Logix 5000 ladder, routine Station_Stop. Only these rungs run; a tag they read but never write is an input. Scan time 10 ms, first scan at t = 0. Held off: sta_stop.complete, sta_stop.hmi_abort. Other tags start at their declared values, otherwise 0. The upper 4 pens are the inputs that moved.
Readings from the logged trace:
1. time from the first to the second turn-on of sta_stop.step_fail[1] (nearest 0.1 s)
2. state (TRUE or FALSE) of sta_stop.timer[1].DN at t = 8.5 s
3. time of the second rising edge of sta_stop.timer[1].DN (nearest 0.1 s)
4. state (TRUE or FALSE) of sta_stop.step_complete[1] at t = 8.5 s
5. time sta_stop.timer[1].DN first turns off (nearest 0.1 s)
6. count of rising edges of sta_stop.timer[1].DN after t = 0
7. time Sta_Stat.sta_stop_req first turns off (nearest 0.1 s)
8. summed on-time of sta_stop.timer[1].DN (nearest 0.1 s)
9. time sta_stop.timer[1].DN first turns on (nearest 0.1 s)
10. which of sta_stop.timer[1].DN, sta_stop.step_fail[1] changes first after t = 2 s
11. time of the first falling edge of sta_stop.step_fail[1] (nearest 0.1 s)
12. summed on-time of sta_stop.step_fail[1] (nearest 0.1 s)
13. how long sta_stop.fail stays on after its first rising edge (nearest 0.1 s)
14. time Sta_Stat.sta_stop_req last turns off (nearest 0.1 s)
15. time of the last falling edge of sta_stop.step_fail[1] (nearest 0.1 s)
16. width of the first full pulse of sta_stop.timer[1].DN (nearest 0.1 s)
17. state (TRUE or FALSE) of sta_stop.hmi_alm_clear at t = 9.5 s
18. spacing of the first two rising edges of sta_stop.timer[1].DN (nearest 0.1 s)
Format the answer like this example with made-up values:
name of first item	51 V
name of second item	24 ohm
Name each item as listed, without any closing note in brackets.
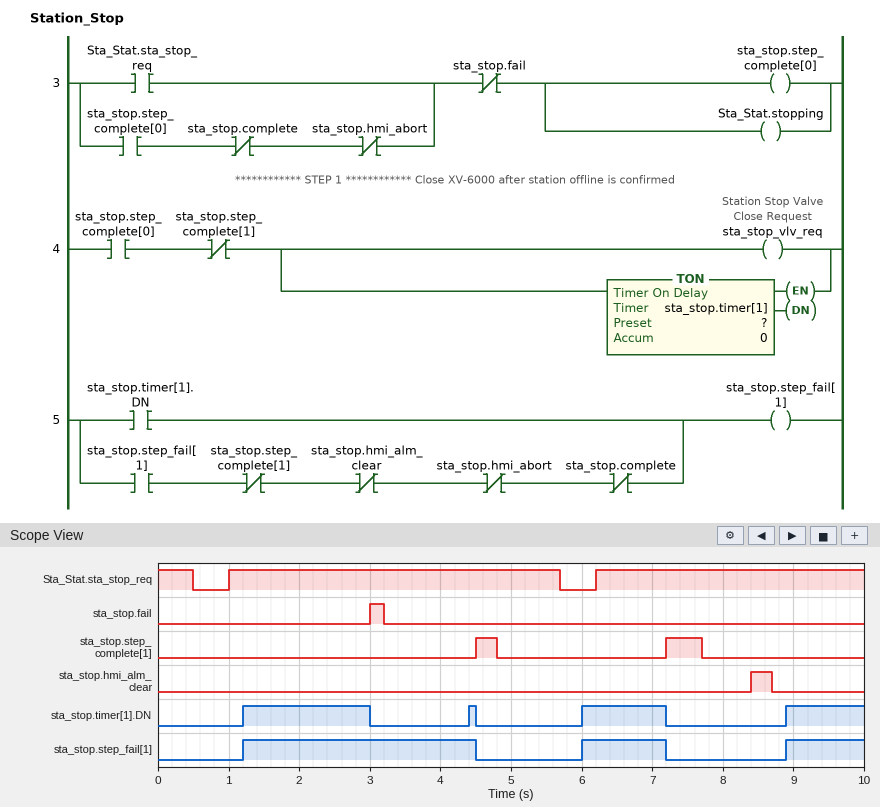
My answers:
time from the first to the second turn-on of sta_stop.step_fail[1]	4.8 s
state (TRUE or FALSE) of sta_stop.timer[1].DN at t = 8.5 s	FALSE
time of the second rising edge of sta_stop.timer[1].DN	4.4 s
state (TRUE or FALSE) of sta_stop.step_complete[1] at t = 8.5 s	FALSE
time sta_stop.timer[1].DN first turns off	3.0 s
count of rising edges of sta_stop.timer[1].DN after t = 0	4
time Sta_Stat.sta_stop_req first turns off	0.5 s
summed on-time of sta_stop.timer[1].DN	4.2 s
time sta_stop.timer[1].DN first turns on	1.2 s
which of sta_stop.timer[1].DN, sta_stop.step_fail[1] changes first after t = 2 s	sta_stop.timer[1].DN
time of the first falling edge of sta_stop.step_fail[1]	4.5 s
summed on-time of sta_stop.step_fail[1]	5.6 s
how long sta_stop.fail stays on after its first rising edge	0.2 s
time Sta_Stat.sta_stop_req last turns off	5.7 s
time of the last falling edge of sta_stop.step_fail[1]	7.2 s
width of the first full pulse of sta_stop.timer[1].DN	1.8 s
state (TRUE or FALSE) of sta_stop.hmi_alm_clear at t = 9.5 s	FALSE
spacing of the first two rising edges of sta_stop.timer[1].DN	3.2 s
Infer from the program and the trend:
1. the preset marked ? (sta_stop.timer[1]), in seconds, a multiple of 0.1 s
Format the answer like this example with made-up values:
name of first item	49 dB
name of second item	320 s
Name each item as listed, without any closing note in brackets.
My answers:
the preset marked ? (sta_stop.timer[1]), in seconds, a multiple of 0.1 s	1.2 s
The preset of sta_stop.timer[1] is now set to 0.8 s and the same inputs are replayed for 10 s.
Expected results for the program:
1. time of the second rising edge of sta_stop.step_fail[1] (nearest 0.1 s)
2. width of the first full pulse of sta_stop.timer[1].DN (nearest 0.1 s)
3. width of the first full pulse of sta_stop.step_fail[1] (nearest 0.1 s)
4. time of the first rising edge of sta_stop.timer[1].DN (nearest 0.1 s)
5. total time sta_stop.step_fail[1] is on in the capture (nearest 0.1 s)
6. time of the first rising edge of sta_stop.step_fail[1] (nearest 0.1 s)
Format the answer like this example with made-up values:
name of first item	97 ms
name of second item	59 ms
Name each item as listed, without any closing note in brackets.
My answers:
time of the second rising edge of sta_stop.step_fail[1]	5.6 s
width of the first full pulse of sta_stop.timer[1].DN	2.2 s
width of the first full pulse of sta_stop.step_fail[1]	3.7 s
time of the first rising edge of sta_stop.timer[1].DN	0.8 s
total time sta_stop.step_fail[1] is on in the capture	6.8 s
time of the first rising edge of sta_stop.step_fail[1]	0.8 s
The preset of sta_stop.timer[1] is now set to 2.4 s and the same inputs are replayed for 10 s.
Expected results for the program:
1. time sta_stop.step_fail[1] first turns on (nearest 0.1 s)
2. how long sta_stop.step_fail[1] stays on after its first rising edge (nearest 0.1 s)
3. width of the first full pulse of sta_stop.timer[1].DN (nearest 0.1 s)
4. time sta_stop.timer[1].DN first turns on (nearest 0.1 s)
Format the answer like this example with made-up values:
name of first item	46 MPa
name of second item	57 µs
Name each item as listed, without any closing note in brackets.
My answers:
time sta_stop.step_fail[1] first turns on	2.4 s
how long sta_stop.step_fail[1] stays on after its first rising edge	2.1 s
width of the first full pulse of sta_stop.timer[1].DN	0.6 s
time sta_stop.timer[1].DN first turns on	2.4 s
